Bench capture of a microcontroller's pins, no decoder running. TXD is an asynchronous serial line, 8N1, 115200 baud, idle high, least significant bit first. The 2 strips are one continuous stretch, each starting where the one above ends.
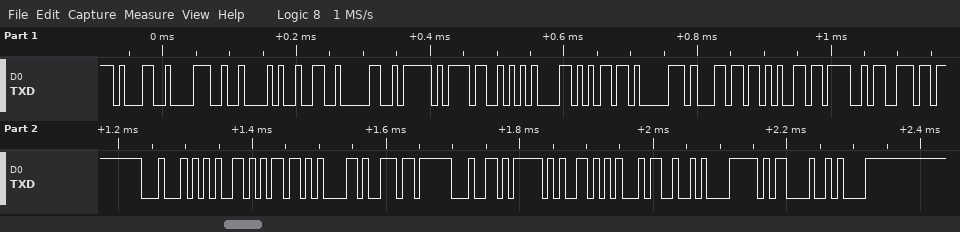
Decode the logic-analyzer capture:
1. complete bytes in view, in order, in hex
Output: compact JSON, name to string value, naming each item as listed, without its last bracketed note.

{"complete bytes in view, in order, in hex": "0x31 0x38 0x42 0x32 0x30 0x5F 0x53 0x61 0x6D 0x70 0x6C 0x65 0x4F 0x6E 0x44 0x65 0x6D 0x61 0x6E 0x64 0x5F 0x56 0x34 0x0A 0x0D 0x0A"}
